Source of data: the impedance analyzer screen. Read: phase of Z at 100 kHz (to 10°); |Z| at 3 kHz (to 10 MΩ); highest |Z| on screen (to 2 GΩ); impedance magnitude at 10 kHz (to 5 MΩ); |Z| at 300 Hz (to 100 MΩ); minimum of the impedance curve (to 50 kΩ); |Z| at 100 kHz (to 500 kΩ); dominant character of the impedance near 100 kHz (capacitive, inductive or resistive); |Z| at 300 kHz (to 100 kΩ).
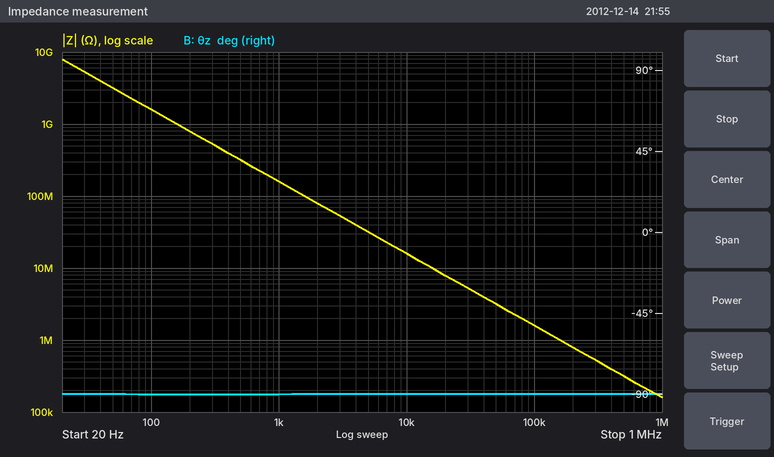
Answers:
-90°
50 MΩ
8 GΩ
15 MΩ
500 MΩ
150 kΩ
1.5 MΩ
capacitive
500 kΩ
